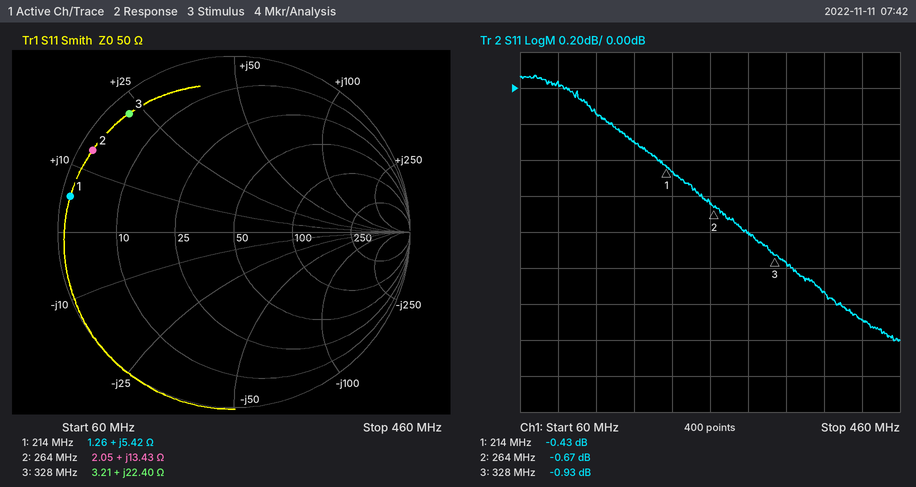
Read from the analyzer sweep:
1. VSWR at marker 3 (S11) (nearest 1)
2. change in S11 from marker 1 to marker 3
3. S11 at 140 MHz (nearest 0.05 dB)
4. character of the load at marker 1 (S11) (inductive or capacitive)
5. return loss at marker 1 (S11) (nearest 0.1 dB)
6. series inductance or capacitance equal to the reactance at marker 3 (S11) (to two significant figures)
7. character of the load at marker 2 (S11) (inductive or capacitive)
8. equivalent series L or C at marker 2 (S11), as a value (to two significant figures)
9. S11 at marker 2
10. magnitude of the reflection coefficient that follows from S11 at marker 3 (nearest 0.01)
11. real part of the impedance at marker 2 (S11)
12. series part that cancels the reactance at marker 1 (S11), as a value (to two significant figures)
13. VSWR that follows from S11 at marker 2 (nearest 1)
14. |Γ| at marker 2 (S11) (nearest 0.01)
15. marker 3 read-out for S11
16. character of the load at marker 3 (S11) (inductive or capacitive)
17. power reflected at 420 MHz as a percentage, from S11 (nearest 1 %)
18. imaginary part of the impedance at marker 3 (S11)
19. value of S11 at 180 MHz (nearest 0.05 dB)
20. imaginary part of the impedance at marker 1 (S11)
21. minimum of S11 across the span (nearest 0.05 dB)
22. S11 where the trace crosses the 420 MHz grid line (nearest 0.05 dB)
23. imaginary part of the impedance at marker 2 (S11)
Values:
19
-0.50 dB
-0.15 dB
inductive
0.4 dB
11 nH
inductive
8.1 nH
-0.67 dB
0.90
2.05 Ω
140 pF
26
0.93
-0.93 dB
inductive
74 %
+22.40 Ω
-0.30 dB
+5.42 Ω
-1.40 dB
-1.30 dB
+13.43 Ω
